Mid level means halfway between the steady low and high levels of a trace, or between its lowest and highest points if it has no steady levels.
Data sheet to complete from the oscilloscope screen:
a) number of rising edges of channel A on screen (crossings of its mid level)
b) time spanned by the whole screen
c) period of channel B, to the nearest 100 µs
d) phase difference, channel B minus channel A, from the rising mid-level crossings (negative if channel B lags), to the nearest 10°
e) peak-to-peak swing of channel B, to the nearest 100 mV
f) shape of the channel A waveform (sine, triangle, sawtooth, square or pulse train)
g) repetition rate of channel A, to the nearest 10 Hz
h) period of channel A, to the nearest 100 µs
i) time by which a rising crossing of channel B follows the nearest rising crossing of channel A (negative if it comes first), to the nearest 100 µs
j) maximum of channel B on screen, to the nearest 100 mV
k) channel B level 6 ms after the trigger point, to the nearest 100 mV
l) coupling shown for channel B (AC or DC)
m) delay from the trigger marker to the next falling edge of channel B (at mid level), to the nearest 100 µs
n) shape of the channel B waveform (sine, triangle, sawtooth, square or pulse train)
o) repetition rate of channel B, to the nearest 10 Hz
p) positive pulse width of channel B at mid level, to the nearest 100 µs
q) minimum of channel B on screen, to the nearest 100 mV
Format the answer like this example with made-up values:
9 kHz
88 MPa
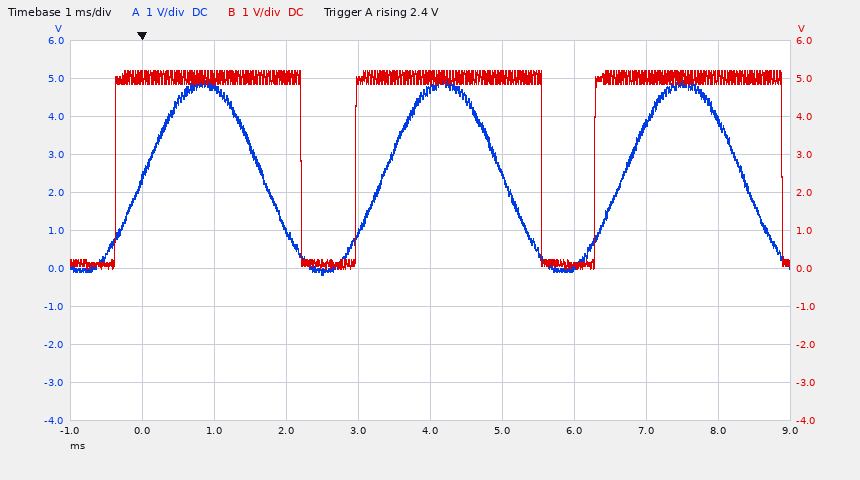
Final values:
3
10 ms
3.3 ms
+40°
5.2 V
sine
300 Hz
3.3 ms
-400 µs
5.2 V
100 mV
DC
2.2 ms
pulse train
300 Hz
2.6 ms
0.0 V
